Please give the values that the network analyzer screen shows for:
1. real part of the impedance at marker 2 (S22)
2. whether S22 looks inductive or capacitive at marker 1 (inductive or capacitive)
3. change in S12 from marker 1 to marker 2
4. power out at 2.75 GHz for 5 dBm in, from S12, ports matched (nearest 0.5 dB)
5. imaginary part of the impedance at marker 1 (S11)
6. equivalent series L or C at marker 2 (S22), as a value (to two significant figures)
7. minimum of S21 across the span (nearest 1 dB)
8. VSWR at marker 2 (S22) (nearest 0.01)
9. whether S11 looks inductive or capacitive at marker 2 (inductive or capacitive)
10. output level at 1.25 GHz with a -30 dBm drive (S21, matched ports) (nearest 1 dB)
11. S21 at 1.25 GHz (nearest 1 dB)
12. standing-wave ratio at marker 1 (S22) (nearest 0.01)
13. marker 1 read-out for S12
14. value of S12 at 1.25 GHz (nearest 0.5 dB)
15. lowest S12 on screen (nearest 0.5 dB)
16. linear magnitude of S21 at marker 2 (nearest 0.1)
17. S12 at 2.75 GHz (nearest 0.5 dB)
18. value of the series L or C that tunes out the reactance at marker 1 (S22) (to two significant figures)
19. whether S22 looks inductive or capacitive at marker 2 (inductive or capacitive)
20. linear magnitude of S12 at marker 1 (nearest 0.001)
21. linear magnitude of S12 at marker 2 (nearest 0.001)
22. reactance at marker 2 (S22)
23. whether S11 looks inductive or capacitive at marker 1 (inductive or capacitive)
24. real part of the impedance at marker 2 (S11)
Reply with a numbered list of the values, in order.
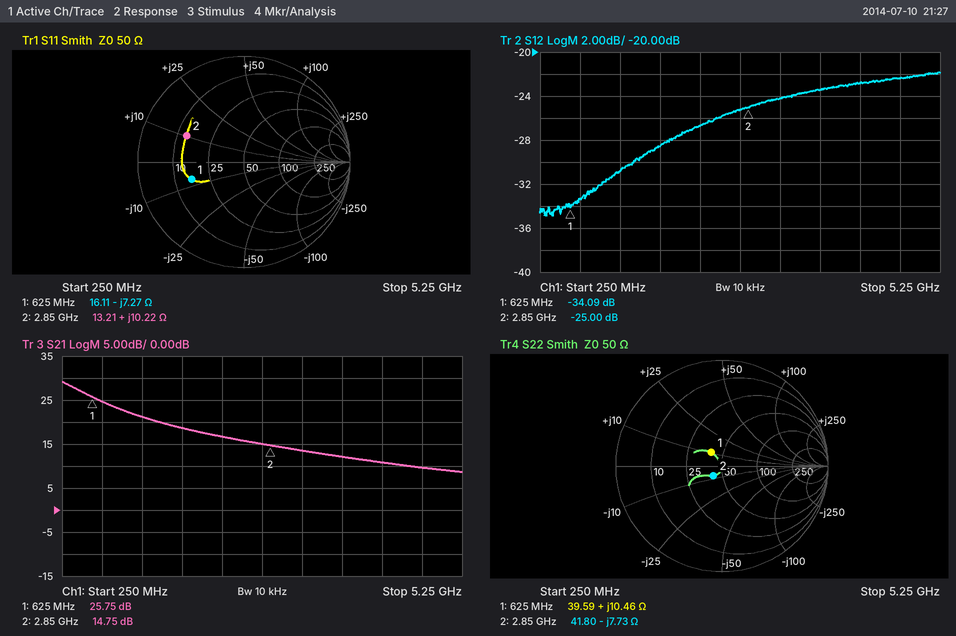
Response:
1. 41.80 Ω
2. inductive
3. 9.09 dB
4. -20.0 dBm
5. -7.27 Ω
6. 7.2 pF
7. 9 dB
8. 1.28
9. inductive
10. -9 dBm
11. 21 dB
12. 1.39
13. -34.09 dB
14. -31.0 dB
15. -35.0 dB
16. 5.5
17. -25.0 dB
18. 24 pF
19. capacitive
20. 0.020
21. 0.056
22. -7.73 Ω
23. capacitive
24. 13.21 Ω
